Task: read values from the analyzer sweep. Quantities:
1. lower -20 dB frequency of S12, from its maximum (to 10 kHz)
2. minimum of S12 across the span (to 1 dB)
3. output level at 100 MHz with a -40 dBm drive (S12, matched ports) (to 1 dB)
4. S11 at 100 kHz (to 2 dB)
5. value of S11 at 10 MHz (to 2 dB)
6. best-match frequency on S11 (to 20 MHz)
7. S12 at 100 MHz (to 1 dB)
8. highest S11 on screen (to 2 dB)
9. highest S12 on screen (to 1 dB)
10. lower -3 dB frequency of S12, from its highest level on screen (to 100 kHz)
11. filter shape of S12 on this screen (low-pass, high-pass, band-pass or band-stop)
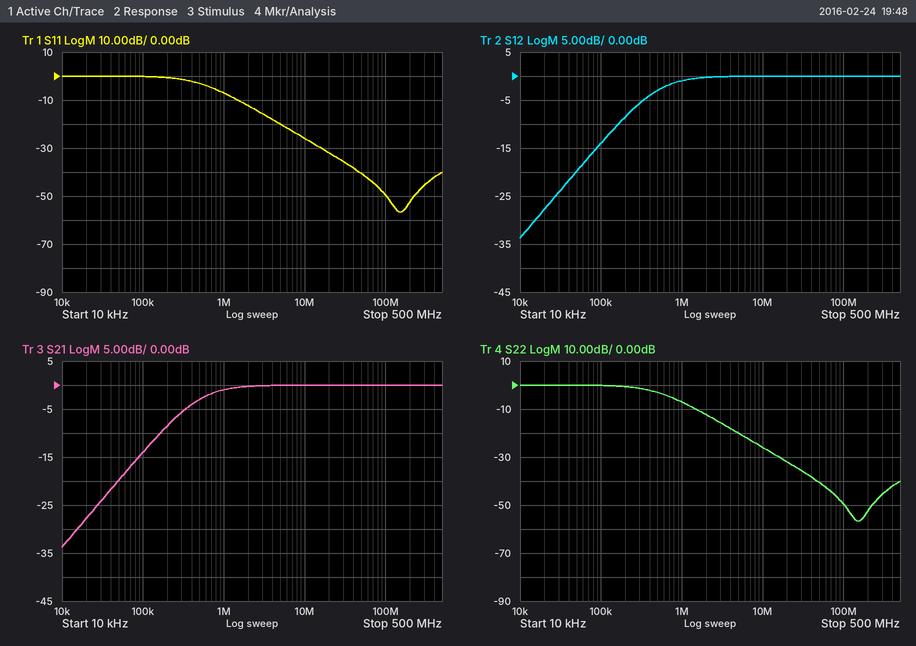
50 kHz
-34 dB
-40 dBm
0 dB
-26 dB
160 MHz
0 dB
0 dB
0 dB
500 kHz
high-pass
